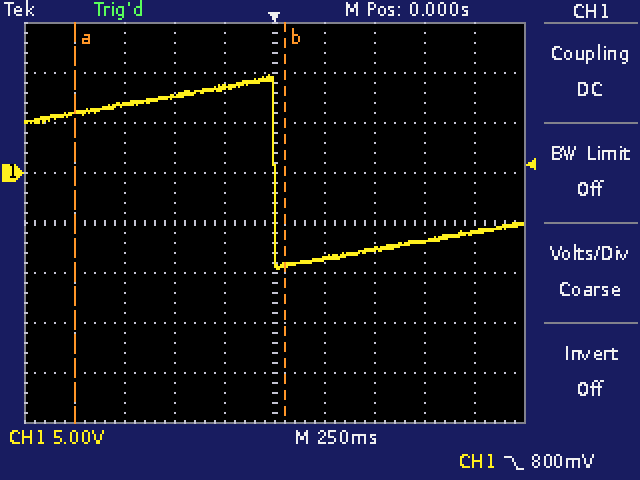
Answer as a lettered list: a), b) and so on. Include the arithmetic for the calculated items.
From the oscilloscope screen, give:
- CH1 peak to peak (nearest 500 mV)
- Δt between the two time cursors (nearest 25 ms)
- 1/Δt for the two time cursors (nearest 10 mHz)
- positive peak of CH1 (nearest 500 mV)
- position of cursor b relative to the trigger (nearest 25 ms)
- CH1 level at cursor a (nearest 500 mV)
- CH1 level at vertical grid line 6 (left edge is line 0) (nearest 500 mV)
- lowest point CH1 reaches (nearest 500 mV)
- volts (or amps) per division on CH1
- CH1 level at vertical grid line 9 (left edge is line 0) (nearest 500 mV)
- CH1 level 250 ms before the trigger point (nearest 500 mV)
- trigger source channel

a) 10.0 V − (-9.5 V) = 19.5 V
b) 1.050 s
c) 1 / 1.050 s ≈ 950 mHz
d) 10.0 V
e) +50 ms
f) 6.0 V
g) -8.5 V
h) -9.5 V
i) 5 V
j) -6.0 V
k) 8.5 V
l) CH1
